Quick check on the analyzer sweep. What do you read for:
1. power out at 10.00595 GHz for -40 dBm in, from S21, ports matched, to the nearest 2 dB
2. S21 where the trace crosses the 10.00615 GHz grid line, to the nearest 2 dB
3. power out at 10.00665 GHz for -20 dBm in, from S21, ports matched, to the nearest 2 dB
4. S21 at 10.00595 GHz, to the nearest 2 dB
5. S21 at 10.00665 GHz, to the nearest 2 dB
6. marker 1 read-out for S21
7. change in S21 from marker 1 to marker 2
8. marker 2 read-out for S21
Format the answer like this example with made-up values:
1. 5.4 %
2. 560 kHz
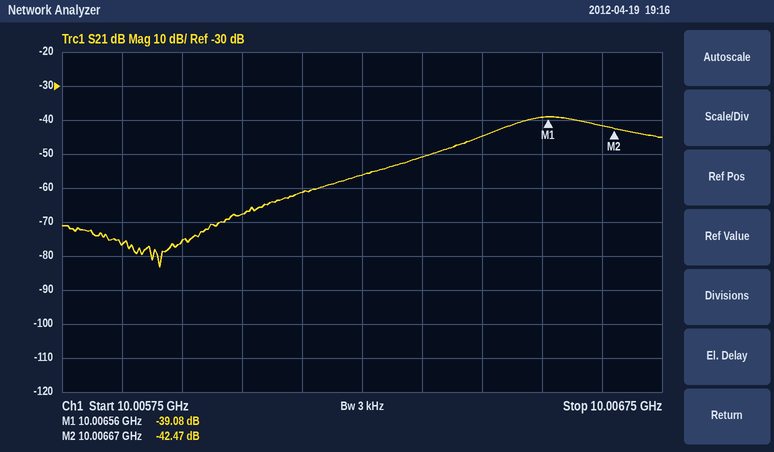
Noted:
1. -116 dBm
2. -62 dB
3. -62 dBm
4. -76 dB
5. -42 dB
6. -39.08 dB
7. -3.39 dB
8. -42.47 dB
